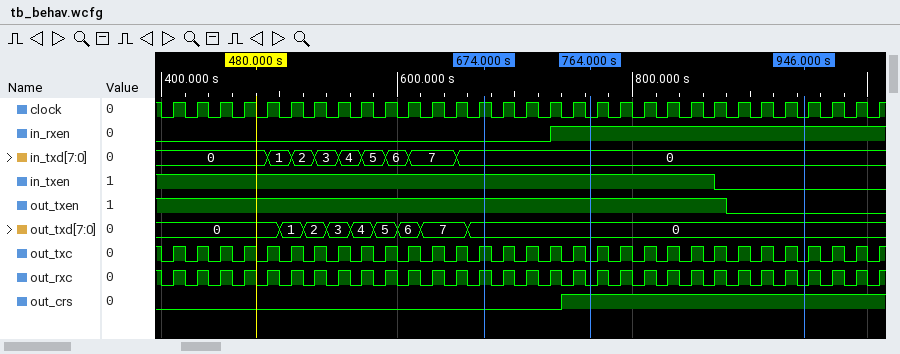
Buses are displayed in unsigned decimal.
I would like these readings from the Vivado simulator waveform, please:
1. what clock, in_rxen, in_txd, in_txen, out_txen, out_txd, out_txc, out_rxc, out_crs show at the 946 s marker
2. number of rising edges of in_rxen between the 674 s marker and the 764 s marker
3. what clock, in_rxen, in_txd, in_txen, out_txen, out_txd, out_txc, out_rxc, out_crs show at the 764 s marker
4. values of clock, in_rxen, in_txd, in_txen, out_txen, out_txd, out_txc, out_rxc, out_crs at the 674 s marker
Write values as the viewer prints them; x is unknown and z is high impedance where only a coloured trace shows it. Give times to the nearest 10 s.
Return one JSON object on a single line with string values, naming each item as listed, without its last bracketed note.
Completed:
{"what clock, in_rxen, in_txd, in_txen, out_txen, out_txd, out_txc, out_rxc, out_crs show at the 946 s marker": "clock=0, in_rxen=1, in_txd=0, in_txen=0, out_txen=0, out_txd=0, out_txc=0, out_rxc=0, out_crs=1", "number of rising edges of in_rxen between the 674 s marker and the 764 s marker": "1", "what clock, in_rxen, in_txd, in_txen, out_txen, out_txd, out_txc, out_rxc, out_crs show at the 764 s marker": "clock=0, in_rxen=1, in_txd=0, in_txen=1, out_txen=1, out_txd=0, out_txc=0, out_rxc=0, out_crs=1", "values of clock, in_rxen, in_txd, in_txen, out_txen, out_txd, out_txc, out_rxc, out_crs at the 674 s marker": "clock=1, in_rxen=0, in_txd=0, in_txen=1, out_txen=1, out_txd=0, out_txc=1, out_rxc=1, out_crs=0"}
